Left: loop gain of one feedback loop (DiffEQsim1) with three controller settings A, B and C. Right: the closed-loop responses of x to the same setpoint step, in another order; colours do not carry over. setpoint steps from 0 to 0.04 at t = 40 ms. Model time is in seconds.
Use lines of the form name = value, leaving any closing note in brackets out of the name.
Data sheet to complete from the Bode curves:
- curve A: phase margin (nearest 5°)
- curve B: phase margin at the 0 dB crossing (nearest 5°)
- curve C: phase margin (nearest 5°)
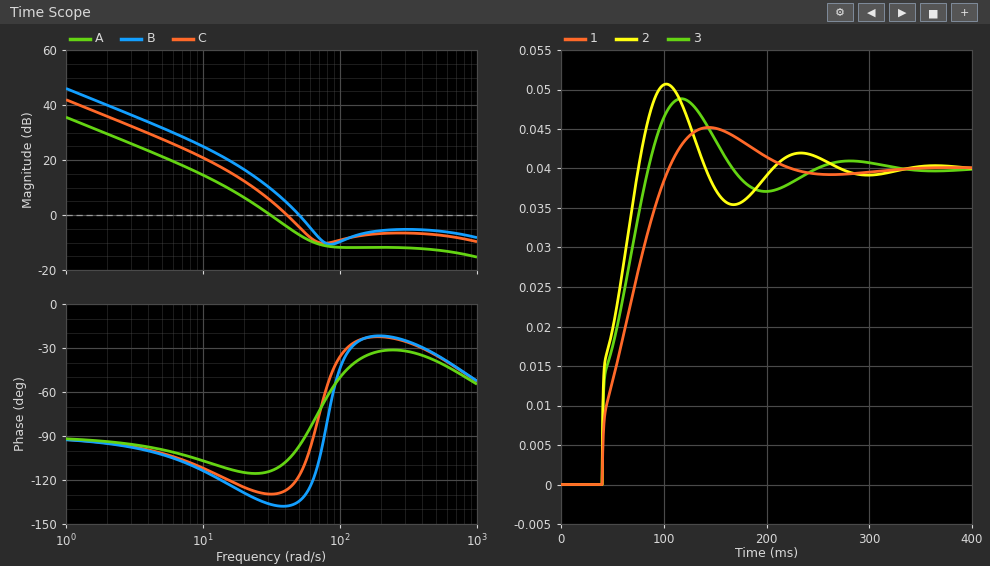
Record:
curve A: phase margin = 65°
curve B: phase margin at the 0 dB crossing = 45°
curve C: phase margin = 55°
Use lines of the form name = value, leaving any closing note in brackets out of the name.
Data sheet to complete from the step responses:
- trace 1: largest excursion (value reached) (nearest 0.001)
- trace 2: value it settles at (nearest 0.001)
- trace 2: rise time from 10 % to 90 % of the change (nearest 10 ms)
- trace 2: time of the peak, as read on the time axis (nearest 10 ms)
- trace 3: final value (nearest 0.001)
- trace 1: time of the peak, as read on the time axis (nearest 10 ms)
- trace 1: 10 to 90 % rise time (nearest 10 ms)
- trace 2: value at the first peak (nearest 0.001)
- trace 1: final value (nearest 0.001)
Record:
trace 1: largest excursion (value reached) = 0.045
trace 2: value it settles at = 0.040
trace 2: rise time from 10 % to 90 % of the change = 30 ms
trace 2: time of the peak, as read on the time axis = 100 ms
trace 3: final value = 0.040
trace 1: time of the peak, as read on the time axis = 140 ms
trace 1: 10 to 90 % rise time = 50 ms
trace 2: value at the first peak = 0.051
trace 1: final value = 0.040
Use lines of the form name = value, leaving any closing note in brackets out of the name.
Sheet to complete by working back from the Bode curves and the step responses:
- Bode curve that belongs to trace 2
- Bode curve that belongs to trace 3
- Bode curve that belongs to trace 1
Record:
Bode curve that belongs to trace 2 = B
Bode curve that belongs to trace 3 = C
Bode curve that belongs to trace 1 = A
